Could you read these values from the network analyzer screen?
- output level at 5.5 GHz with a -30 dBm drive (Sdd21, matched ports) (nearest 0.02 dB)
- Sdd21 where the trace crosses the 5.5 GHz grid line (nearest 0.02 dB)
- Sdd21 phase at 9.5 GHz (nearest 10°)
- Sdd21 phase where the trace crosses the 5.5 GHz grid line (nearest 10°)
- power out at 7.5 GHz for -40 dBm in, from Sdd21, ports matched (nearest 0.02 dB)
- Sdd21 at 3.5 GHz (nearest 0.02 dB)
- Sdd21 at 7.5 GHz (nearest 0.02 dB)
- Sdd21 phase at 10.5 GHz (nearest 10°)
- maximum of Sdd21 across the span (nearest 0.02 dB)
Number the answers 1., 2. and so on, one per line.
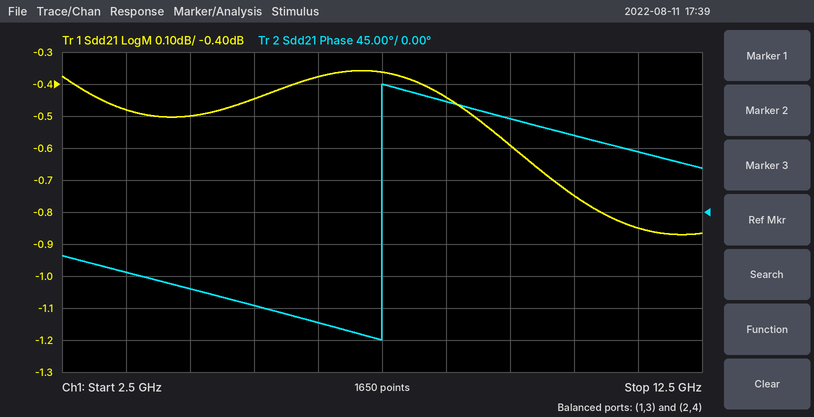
1. -30.44 dBm
2. -0.44 dB
3. 130°
4. -130°
5. -40.36 dBm
6. -0.48 dB
7. -0.36 dB
8. 110°
9. -0.36 dB
